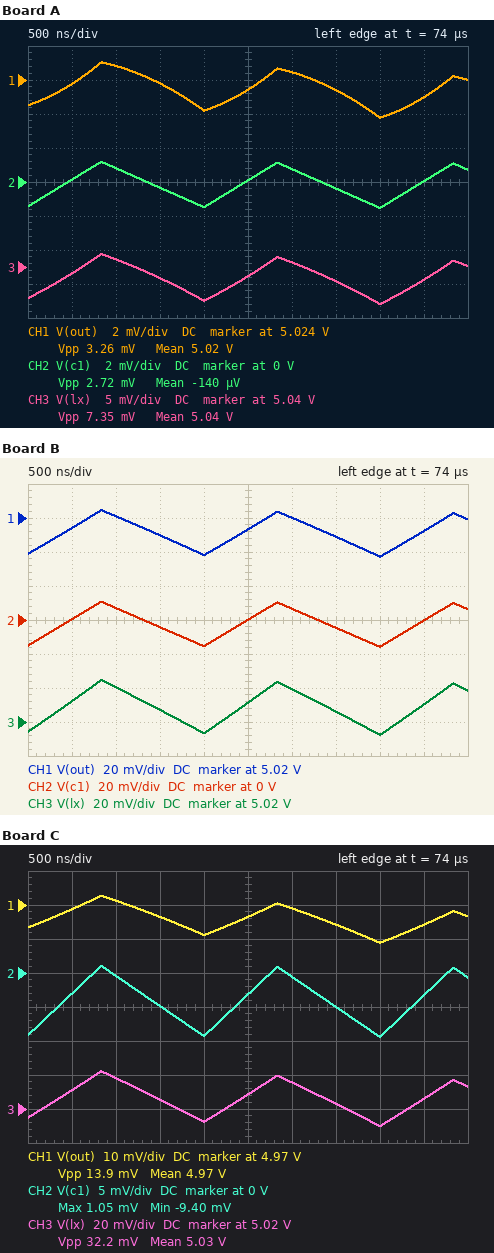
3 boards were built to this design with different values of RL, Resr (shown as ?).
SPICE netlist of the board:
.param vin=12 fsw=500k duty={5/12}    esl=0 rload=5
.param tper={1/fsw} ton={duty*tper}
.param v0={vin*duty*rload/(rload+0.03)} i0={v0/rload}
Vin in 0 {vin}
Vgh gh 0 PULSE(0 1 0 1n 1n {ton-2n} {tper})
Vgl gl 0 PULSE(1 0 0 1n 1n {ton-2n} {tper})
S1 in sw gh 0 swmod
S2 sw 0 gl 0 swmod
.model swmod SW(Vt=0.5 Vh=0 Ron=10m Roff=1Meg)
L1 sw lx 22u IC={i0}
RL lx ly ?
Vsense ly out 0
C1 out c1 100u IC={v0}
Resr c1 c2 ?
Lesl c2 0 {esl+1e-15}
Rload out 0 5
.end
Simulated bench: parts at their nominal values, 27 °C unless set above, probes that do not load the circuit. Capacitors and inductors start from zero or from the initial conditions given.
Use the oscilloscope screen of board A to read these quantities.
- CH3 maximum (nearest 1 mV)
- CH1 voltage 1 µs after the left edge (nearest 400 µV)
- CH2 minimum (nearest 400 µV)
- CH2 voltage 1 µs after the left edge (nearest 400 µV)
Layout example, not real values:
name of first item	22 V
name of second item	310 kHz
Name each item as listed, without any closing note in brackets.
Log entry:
CH3 maximum	5.042 V
CH1 voltage 1 µs after the left edge	5.0248 V
CH2 minimum	-1.6 mV
CH2 voltage 1 µs after the left edge	800 µV
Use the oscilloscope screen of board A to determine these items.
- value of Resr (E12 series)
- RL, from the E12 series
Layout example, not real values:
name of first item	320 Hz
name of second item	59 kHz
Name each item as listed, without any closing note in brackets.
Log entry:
value of Resr	0.01 Ω
RL, from the E12 series	0.015 Ω
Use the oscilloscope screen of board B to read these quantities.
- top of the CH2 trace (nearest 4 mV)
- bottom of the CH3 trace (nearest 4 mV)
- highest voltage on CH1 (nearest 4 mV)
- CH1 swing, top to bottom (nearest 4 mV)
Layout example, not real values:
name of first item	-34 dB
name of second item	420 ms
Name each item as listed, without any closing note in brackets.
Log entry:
top of the CH2 trace	12 mV
bottom of the CH3 trace	5.012 V
highest voltage on CH1	5.024 V
CH1 swing, top to bottom	28 mV
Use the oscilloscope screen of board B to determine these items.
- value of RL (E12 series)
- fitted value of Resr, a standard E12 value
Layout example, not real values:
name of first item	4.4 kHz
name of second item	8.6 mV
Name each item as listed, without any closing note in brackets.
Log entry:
value of RL	0.018 Ω
fitted value of Resr, a standard E12 value	0.1 Ω
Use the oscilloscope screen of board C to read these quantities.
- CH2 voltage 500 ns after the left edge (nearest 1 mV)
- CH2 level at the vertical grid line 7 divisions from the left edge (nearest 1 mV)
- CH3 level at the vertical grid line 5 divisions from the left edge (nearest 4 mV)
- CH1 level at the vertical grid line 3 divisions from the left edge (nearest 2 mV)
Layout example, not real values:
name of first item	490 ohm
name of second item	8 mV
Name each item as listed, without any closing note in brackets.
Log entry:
CH2 voltage 500 ns after the left edge	-3 mV
CH2 level at the vertical grid line 7 divisions from the left edge	-5 mV
CH3 level at the vertical grid line 5 divisions from the left edge	5.028 V
CH1 level at the vertical grid line 3 divisions from the left edge	4.966 V
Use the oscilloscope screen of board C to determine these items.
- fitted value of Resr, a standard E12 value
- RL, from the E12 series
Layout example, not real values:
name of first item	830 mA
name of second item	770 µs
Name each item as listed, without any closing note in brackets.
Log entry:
fitted value of Resr, a standard E12 value	0.039 Ω
RL, from the E12 series	0.068 Ω
